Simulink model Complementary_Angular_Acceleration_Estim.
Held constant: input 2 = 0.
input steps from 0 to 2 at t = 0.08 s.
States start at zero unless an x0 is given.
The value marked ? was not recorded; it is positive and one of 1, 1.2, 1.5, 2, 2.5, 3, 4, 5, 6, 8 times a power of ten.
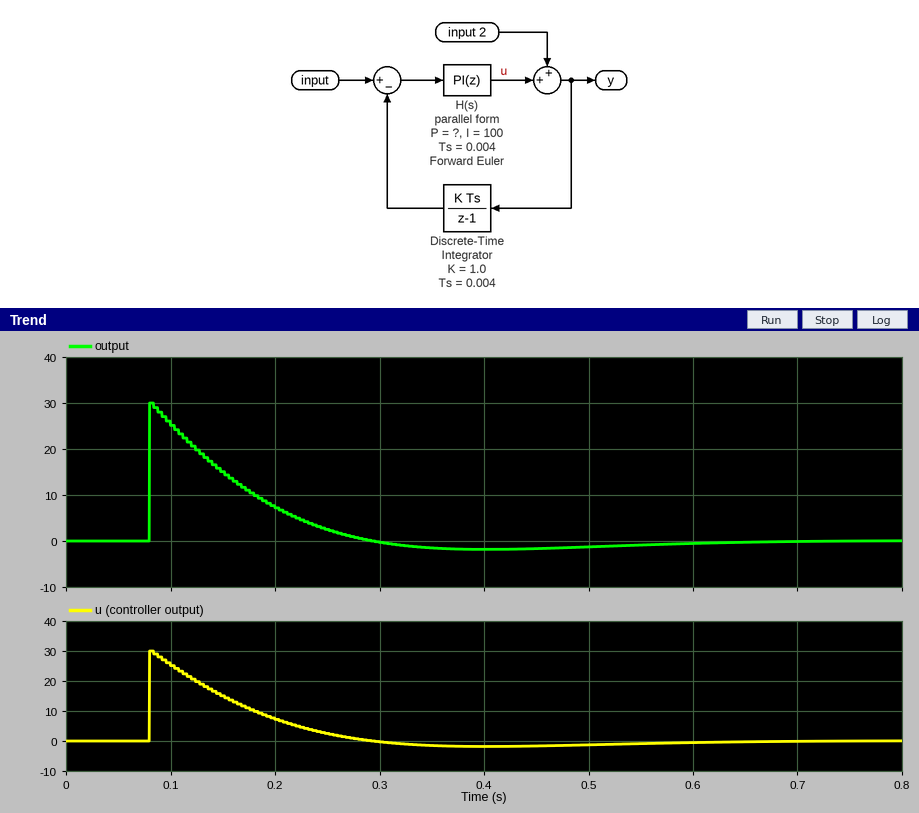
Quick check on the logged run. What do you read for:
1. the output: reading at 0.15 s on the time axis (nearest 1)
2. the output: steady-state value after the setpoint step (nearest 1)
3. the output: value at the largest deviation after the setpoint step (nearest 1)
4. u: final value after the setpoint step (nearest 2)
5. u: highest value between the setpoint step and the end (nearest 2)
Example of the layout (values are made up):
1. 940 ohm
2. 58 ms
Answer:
1. 15
2. 0
3. 30
4. 0
5. 30
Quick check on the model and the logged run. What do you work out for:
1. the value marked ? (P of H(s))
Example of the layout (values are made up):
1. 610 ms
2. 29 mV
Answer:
1. 15
